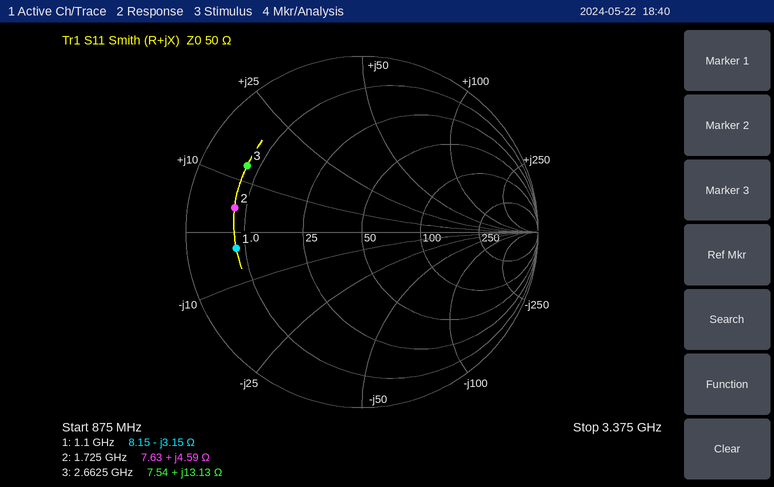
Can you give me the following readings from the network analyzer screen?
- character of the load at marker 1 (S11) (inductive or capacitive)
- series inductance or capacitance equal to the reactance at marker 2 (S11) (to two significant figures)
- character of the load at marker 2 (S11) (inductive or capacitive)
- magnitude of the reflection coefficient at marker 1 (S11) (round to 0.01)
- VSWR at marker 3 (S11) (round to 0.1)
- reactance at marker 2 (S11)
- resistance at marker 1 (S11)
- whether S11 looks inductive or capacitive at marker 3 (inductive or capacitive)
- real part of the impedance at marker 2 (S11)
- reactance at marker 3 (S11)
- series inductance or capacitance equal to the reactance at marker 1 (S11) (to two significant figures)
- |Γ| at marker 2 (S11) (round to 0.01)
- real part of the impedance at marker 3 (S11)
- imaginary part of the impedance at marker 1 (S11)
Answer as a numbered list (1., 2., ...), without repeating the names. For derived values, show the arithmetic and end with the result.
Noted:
1. capacitive
2. L = 4.59 Ω/(2π × 1.725 GHz) ≈ 423 pH, so 420 pH to two significant figures
3. inductive
4. 0.72
5. 7.1
6. +4.59 Ω
7. 8.15 Ω
8. inductive
9. 7.63 Ω
10. +13.13 Ω
11. C = 1/(2π × 1.1 GHz × 3.15 Ω) ≈ 46 pF
12. 0.74
13. 7.54 Ω
14. -3.15 Ω
